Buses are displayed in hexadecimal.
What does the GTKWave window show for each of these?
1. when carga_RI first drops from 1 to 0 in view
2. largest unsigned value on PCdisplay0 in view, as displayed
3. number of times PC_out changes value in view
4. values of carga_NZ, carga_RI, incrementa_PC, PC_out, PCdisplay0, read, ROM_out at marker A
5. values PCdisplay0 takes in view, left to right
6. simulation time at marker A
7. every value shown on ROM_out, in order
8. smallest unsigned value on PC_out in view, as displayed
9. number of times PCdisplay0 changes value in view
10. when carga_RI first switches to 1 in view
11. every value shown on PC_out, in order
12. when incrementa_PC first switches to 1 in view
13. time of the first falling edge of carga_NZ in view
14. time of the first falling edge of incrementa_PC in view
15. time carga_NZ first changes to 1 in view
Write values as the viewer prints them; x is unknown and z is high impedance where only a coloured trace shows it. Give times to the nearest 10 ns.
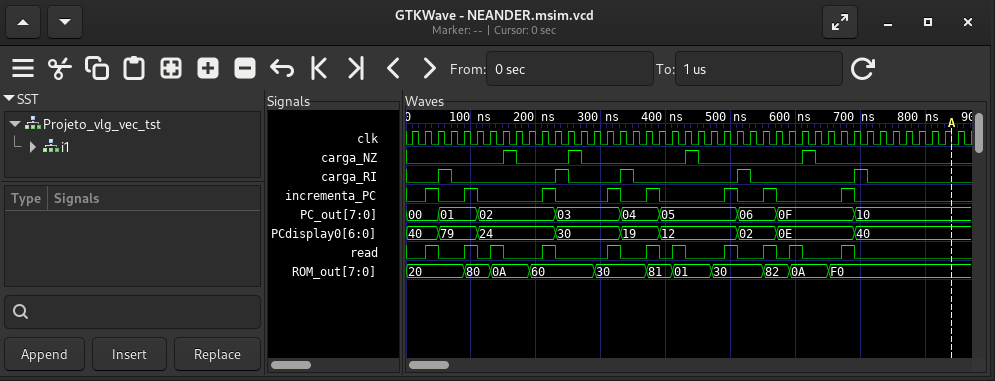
70 ns
79
8
carga_NZ=0, carga_RI=0, incrementa_PC=0, PC_out=10, PCdisplay0=40, read=0, ROM_out=F0
40, 79, 24, 30, 19, 12, 02, 0E, 40
840 ns
20, 80, 0A, 60, 30, 81, 01, 30, 82, 0A, F0
00
8
50 ns
00, 01, 02, 03, 04, 05, 06, 0F, 10
30 ns
170 ns
50 ns
150 ns
